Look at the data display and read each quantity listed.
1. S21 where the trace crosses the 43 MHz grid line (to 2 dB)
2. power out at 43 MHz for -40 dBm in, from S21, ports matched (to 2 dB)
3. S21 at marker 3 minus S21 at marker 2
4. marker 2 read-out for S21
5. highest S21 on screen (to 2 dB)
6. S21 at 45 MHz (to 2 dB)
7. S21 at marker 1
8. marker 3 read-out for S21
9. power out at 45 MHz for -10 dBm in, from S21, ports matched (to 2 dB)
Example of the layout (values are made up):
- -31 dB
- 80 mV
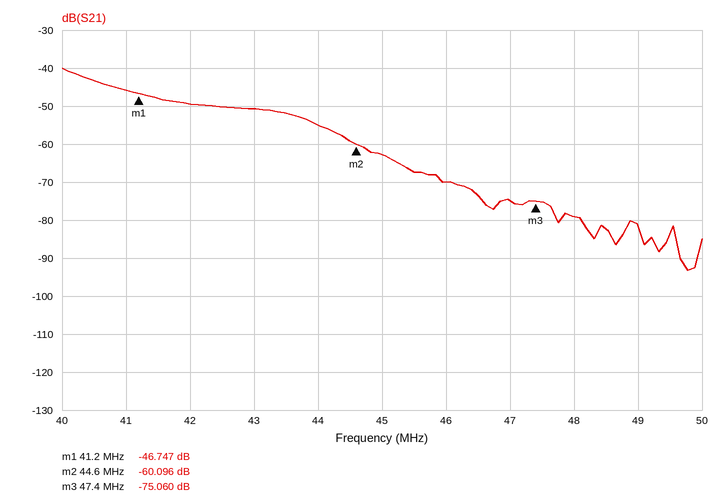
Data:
- -50 dB
- -90 dBm
- -14.964 dB
- -60.096 dB
- -40 dB
- -62 dB
- -46.747 dB
- -75.060 dB
- -72 dBm
